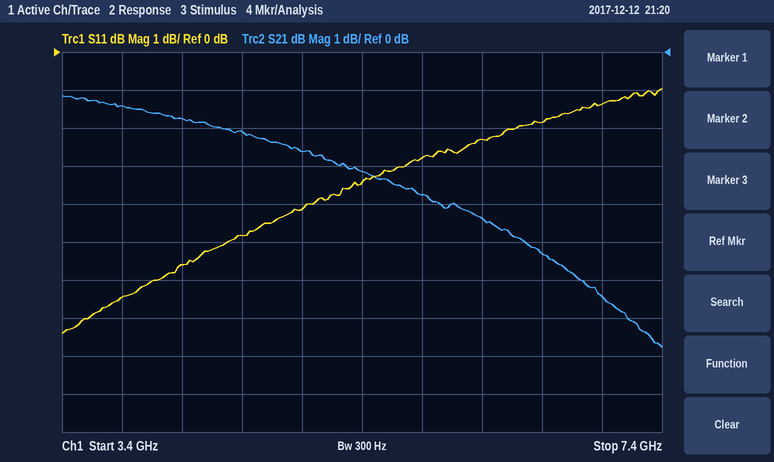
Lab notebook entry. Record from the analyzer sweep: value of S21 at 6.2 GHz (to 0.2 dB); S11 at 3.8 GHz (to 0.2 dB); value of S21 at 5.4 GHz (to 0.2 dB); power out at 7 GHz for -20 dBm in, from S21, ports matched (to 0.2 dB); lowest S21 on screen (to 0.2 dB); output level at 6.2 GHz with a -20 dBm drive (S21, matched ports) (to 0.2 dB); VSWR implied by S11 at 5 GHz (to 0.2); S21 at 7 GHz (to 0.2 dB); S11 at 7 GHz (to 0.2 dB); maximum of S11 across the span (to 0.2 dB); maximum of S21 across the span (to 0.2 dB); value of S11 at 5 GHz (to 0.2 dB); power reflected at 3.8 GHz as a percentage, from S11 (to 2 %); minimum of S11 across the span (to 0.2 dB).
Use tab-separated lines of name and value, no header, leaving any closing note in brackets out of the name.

value of S21 at 6.2 GHz	-4.4 dB
S11 at 3.8 GHz	-6.4 dB
value of S21 at 5.4 GHz	-3.2 dB
power out at 7 GHz for -20 dBm in, from S21, ports matched	-26.4 dBm
lowest S21 on screen	-7.8 dB
output level at 6.2 GHz with a -20 dBm drive (S21, matched ports)	-24.4 dBm
VSWR implied by S11 at 5 GHz	4.2
S21 at 7 GHz	-6.4 dB
S11 at 7 GHz	-1.4 dB
maximum of S11 across the span	-1.0 dB
maximum of S21 across the span	-1.2 dB
value of S11 at 5 GHz	-4.2 dB
power reflected at 3.8 GHz as a percentage, from S11	22 %
minimum of S11 across the span	-7.4 dB
